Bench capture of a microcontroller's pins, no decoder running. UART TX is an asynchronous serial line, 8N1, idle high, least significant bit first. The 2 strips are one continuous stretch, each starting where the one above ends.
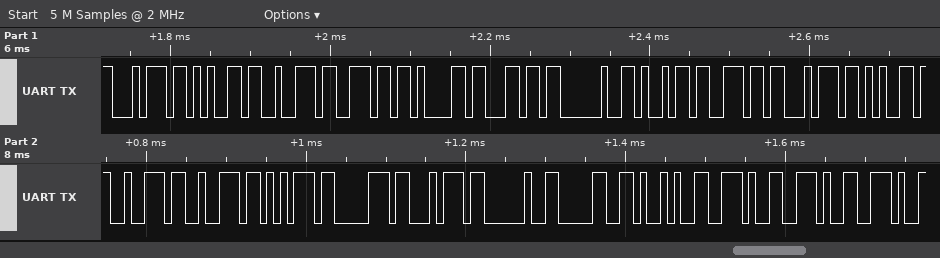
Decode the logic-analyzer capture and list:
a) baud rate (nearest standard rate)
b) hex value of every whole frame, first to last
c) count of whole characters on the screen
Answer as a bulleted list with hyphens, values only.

- 115200 baud
- 74 65 72 6E 61 6C 20 69 6E 74 65 72 72 75 70 74 20 30 29 2E 2E 2E
- 22
